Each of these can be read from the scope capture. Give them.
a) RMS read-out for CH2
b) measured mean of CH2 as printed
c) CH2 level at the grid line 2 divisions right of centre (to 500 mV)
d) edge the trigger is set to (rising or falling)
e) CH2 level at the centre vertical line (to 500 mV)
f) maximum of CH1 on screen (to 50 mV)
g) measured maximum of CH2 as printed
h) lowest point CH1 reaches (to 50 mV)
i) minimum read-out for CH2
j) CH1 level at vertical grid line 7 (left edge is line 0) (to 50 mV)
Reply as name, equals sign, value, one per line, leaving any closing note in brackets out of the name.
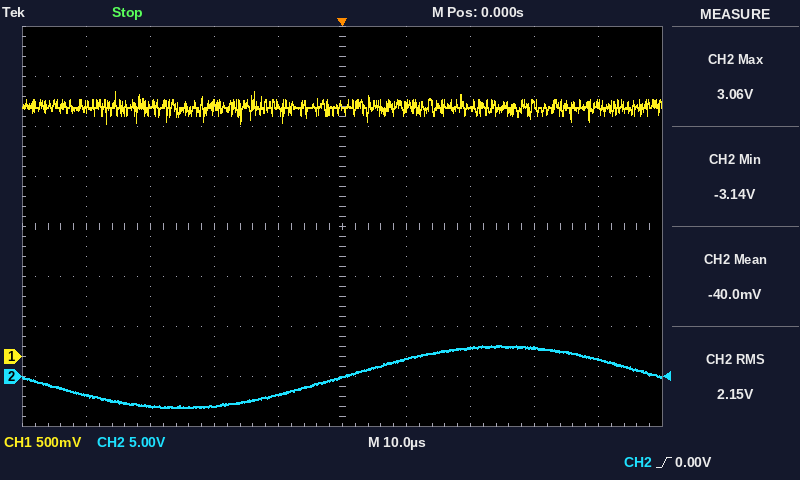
RMS read-out for CH2 = 2.15 V
measured mean of CH2 as printed = -40.0 mV
CH2 level at the grid line 2 divisions right of centre = 3.0 V
edge the trigger is set to = rising
CH2 level at the centre vertical line = 0.0 V
maximum of CH1 on screen = 2.65 V
measured maximum of CH2 as printed = 3.06 V
lowest point CH1 reaches = 2.35 V
minimum read-out for CH2 = -3.14 V
CH1 level at vertical grid line 7 (left edge is line 0) = 2.50 V
